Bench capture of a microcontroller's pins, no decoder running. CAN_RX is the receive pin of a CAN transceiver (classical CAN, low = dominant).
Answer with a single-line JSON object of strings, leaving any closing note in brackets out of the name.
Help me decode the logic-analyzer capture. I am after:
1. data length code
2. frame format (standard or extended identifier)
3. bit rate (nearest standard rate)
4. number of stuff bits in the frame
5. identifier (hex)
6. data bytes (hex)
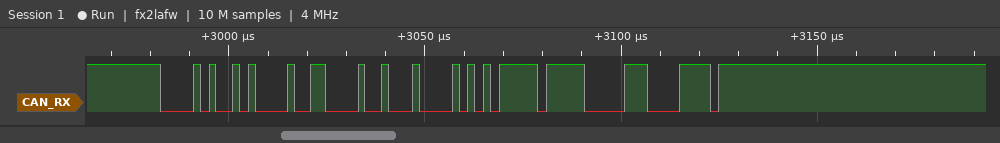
{"data length code": "4", "frame format": "standard", "bit rate": "500 kbit/s", "number of stuff bits in the frame": "3", "identifier": "0x0A5", "data bytes": "C2 44 2A FF"}
